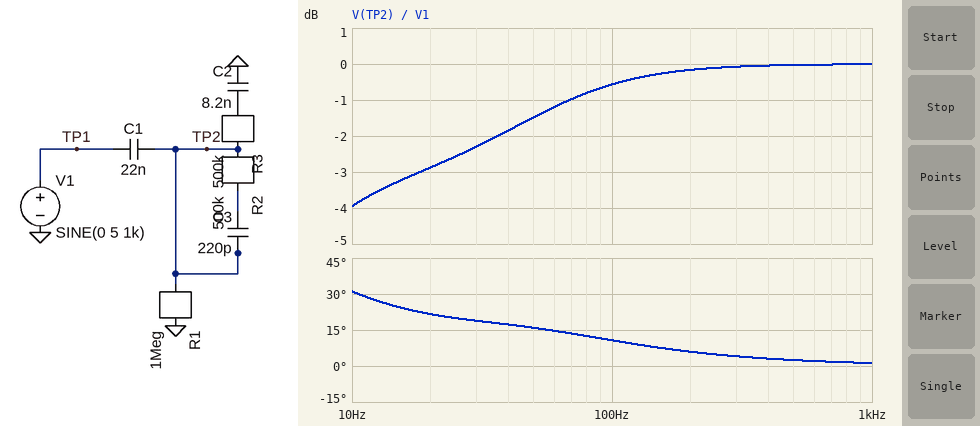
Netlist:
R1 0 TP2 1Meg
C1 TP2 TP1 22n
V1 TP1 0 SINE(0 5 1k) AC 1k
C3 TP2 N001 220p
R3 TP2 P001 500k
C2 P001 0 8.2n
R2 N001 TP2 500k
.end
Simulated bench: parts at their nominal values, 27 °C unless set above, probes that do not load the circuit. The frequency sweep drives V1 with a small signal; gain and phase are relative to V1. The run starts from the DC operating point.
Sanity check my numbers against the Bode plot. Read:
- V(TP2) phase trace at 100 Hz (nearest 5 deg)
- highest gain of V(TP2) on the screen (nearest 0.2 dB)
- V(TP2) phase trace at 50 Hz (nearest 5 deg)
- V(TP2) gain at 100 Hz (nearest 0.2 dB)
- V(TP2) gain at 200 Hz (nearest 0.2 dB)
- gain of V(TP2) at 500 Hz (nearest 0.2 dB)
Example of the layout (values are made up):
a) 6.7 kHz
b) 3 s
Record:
a) 10 deg
b) 0 dB
c) 15 deg
d) -0.6 dB
e) -0.2 dB
f) 0 dB
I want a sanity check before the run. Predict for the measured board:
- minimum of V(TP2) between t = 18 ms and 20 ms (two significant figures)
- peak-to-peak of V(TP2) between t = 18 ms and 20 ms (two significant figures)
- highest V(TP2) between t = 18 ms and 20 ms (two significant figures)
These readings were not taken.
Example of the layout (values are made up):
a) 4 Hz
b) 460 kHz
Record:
a) -5.0 V
b) 10 V
c) 5.0 V
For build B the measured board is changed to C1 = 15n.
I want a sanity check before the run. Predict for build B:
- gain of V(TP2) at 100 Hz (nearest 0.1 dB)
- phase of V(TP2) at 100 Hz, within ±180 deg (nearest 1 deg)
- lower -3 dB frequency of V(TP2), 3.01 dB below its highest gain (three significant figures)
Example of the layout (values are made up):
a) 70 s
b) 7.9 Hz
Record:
a) -0.9 dB
b) 15 deg
c) 35.9 Hz
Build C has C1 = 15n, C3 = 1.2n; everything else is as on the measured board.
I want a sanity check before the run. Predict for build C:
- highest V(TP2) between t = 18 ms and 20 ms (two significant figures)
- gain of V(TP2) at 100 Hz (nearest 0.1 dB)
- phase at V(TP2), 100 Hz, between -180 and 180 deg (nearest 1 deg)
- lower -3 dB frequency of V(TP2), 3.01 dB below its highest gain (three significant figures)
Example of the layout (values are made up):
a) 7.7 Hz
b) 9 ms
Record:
a) 5.0 V
b) -0.9 dB
c) 15 deg
d) 35.9 Hz
